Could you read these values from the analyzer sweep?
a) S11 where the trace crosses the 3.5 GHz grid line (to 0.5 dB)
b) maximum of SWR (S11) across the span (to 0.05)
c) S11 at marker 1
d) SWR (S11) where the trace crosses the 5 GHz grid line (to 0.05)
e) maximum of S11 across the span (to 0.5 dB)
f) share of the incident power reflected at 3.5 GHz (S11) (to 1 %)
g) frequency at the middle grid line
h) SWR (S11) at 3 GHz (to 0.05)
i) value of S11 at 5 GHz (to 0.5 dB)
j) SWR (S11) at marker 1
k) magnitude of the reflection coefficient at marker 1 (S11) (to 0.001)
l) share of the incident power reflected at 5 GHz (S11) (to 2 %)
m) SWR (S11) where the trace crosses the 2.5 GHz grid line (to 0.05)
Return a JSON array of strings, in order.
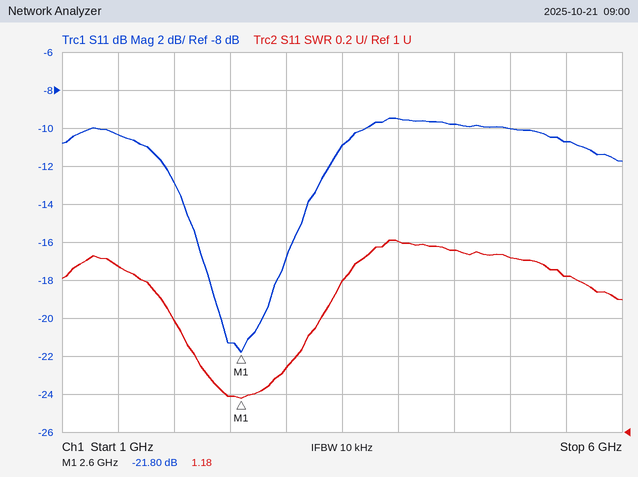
["-11.0 dB", "2.00", "-21.80 dB", "1.90", "-9.5 dB", "8 %", "3.5 GHz", "1.35", "-10.0 dB", "1.18", "0.081", "10 %", "1.20"]
